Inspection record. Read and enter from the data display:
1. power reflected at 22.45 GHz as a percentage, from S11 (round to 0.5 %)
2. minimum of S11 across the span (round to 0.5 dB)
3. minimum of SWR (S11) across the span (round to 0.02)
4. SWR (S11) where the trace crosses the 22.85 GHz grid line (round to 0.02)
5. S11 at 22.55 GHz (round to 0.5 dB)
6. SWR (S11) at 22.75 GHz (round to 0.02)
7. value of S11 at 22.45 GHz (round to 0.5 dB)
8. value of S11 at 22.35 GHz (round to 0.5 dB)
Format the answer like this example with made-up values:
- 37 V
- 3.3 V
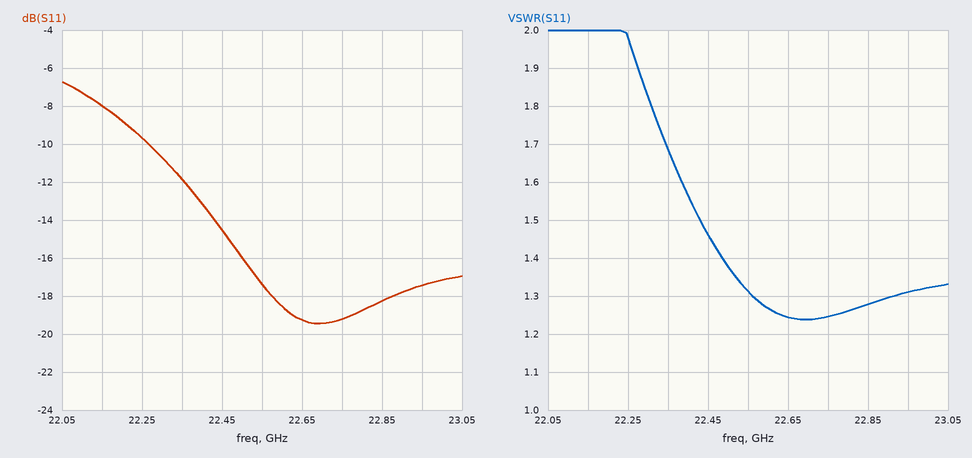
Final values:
- 3.5 %
- -19.5 dB
- 1.24
- 1.28
- -17.5 dB
- 1.24
- -14.5 dB
- -12.0 dB
